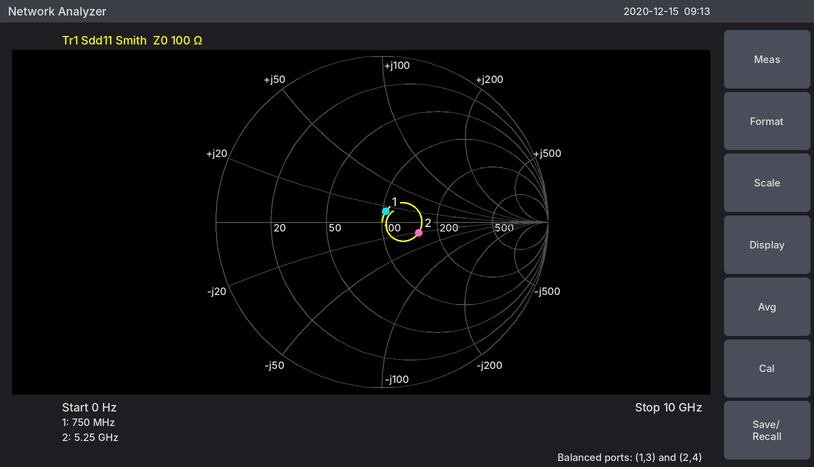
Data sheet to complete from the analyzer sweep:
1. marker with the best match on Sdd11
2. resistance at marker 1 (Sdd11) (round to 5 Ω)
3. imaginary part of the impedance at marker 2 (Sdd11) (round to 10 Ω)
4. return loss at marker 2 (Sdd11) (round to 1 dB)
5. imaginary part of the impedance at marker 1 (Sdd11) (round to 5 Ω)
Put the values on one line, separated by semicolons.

marker 1; 105 Ω; -20 Ω; 13 dB; +15 Ω
